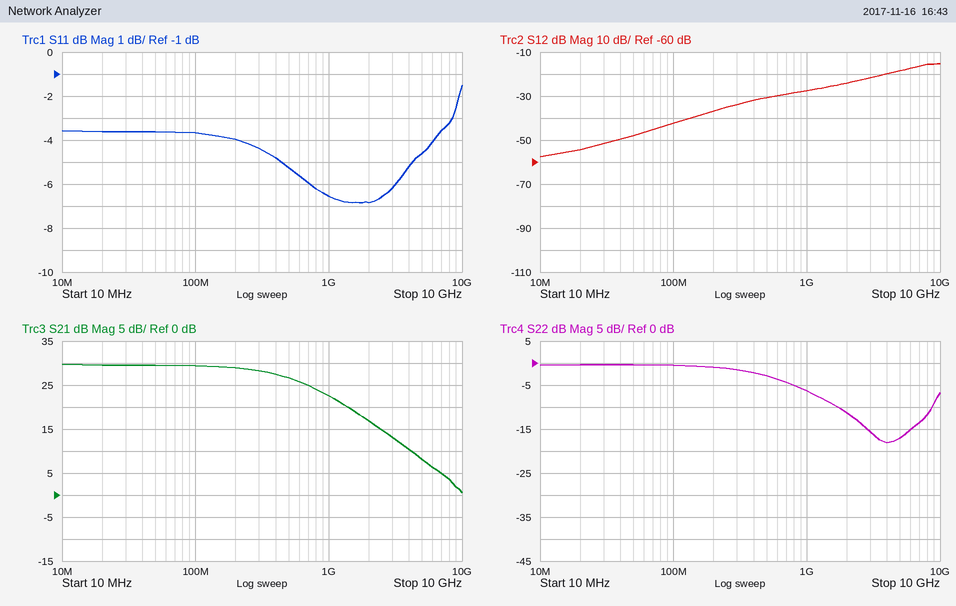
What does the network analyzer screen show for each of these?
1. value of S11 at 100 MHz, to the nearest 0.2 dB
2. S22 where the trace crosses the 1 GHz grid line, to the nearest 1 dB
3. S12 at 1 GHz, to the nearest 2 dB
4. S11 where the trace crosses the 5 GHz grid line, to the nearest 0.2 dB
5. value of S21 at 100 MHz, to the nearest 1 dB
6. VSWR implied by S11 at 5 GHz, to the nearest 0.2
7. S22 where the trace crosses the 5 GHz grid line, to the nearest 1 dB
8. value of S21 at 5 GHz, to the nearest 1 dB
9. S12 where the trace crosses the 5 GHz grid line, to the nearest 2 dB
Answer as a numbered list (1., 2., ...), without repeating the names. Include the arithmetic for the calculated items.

1. -3.6 dB
2. -6 dB
3. -28 dB
4. -4.6 dB
5. 29 dB
6. |Γ| = 10^(-4.6/20) = 0.5888; VSWR = (1 + 0.5888)/(1 − 0.5888) ≈ 3.86, so 3.8 to the nearest 0.2
7. -17 dB
8. 8 dB
9. -18 dB
